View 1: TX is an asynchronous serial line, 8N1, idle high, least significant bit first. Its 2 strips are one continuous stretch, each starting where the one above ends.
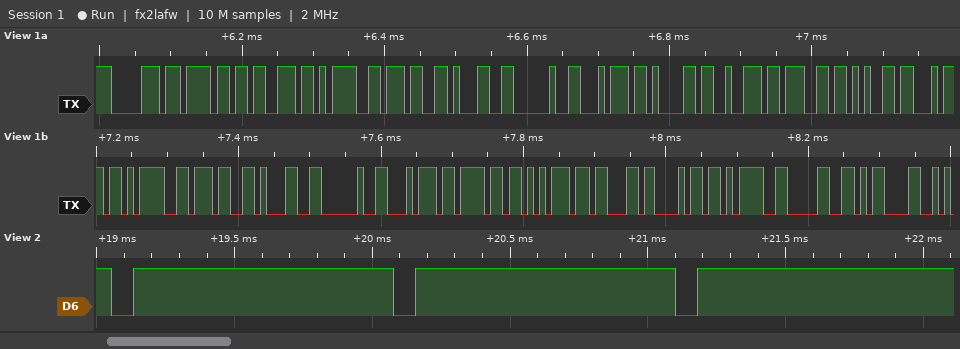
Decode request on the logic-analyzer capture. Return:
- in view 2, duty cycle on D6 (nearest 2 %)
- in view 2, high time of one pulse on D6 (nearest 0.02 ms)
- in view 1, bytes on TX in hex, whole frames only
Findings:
92 %
0.94 ms
0x70 0x6F 0x73 0x3D 0x37 0x31 0x20 0x74 0x61 0x72 0x67 0x65 0x74 0x3D 0x37 0x31 0x20 0x74 0x6F 0x75 0x63 0x68 0x3D 0x30 0x0D
